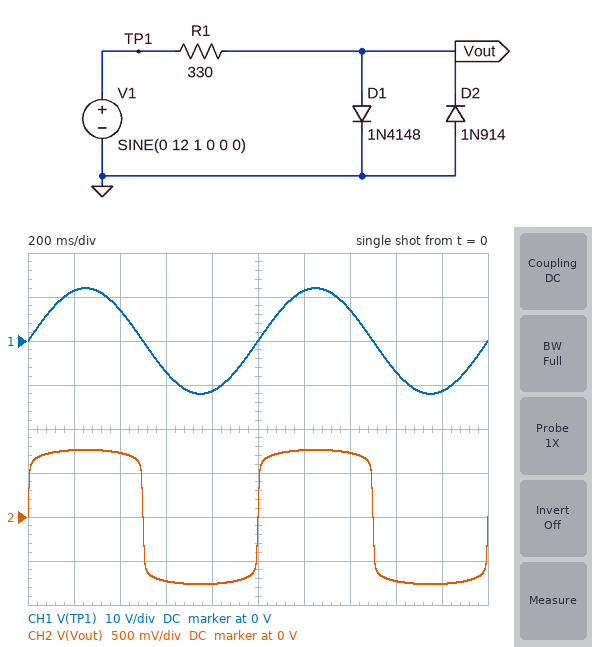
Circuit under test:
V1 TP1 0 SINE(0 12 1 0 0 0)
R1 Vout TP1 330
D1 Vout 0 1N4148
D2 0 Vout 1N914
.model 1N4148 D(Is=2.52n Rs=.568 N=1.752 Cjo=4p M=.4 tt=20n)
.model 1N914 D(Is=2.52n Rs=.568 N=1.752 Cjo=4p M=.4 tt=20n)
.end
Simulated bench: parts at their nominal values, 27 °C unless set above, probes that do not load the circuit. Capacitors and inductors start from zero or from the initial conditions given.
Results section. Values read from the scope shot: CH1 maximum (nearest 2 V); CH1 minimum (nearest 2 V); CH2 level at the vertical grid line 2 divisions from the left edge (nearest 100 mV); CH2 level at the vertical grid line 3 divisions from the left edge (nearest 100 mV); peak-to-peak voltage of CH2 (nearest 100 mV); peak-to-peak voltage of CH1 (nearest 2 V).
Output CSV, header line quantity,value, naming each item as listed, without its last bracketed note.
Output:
quantity,value
CH1 maximum,12 V
CH1 minimum,-12 V
CH2 level at the vertical grid line 2 divisions from the left edge,700 mV
CH2 level at the vertical grid line 3 divisions from the left edge,-700 mV
peak-to-peak voltage of CH2,1.5 V
peak-to-peak voltage of CH1,24 V
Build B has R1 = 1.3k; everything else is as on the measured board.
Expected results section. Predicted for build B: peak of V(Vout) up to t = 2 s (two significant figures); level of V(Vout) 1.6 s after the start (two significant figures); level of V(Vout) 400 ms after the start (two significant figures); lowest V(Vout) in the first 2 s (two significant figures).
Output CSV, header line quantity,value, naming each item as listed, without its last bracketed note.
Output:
quantity,value
peak of V(Vout) up to t = 2 s,690 mV
level of V(Vout) 1.6 s after the start,-660 mV
level of V(Vout) 400 ms after the start,660 mV
lowest V(Vout) in the first 2 s,-690 mV
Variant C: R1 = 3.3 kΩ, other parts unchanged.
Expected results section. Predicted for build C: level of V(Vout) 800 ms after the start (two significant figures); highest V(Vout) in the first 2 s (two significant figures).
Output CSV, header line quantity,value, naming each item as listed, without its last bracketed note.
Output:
quantity,value
level of V(Vout) 800 ms after the start,-640 mV
highest V(Vout) in the first 2 s,640 mV
